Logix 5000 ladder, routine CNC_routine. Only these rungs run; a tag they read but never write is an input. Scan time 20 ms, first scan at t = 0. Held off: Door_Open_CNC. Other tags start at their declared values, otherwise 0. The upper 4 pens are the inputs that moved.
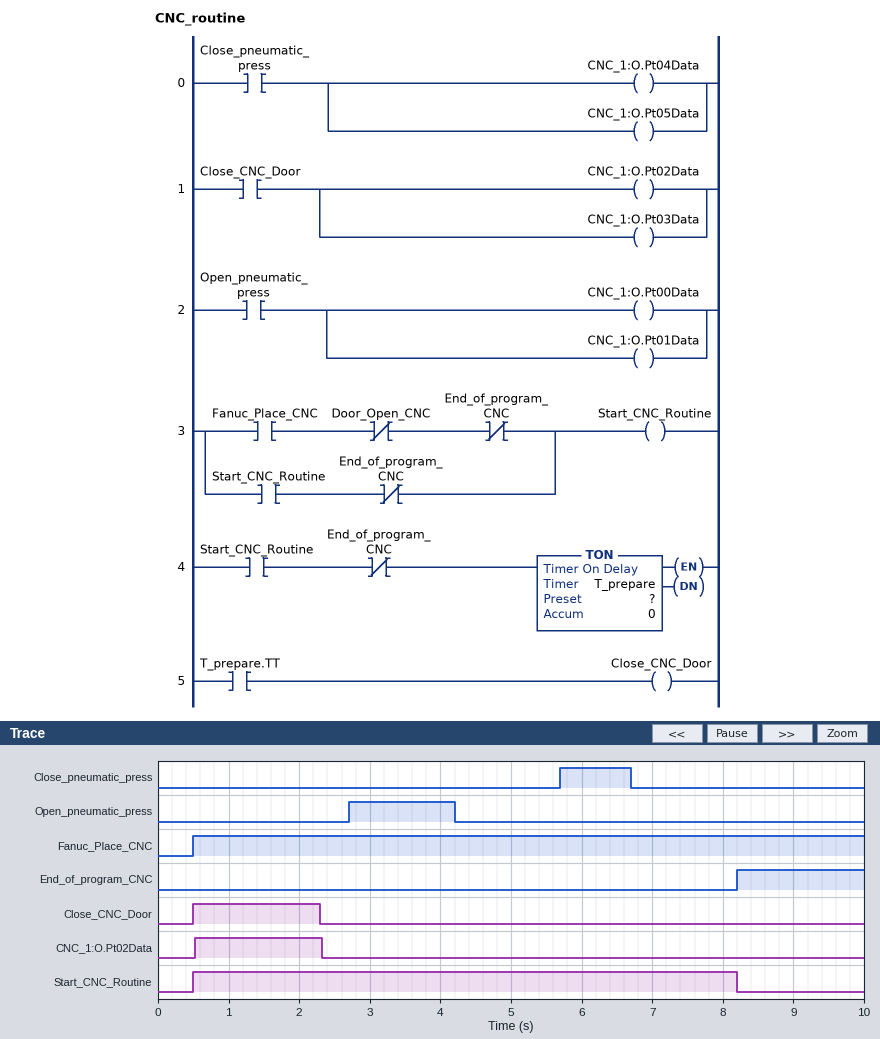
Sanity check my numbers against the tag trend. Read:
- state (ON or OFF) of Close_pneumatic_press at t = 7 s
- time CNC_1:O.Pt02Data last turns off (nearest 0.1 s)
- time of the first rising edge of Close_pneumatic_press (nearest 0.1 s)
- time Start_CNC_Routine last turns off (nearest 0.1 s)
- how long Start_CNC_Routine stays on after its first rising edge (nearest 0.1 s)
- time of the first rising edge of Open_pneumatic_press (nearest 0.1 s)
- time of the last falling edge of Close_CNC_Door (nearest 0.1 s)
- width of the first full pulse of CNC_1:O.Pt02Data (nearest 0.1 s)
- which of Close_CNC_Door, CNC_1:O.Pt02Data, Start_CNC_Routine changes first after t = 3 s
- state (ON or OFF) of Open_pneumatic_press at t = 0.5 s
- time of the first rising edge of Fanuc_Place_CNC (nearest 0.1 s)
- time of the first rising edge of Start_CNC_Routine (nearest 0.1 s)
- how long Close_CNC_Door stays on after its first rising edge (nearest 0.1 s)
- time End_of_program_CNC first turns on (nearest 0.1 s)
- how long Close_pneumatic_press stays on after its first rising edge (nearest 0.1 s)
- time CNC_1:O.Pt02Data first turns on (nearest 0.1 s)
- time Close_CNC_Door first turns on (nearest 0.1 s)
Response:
OFF
2.3 s
5.7 s
8.2 s
7.7 s
2.7 s
2.3 s
1.8 s
Start_CNC_Routine
OFF
0.5 s
0.5 s
1.8 s
8.2 s
1.0 s
0.5 s
0.5 s
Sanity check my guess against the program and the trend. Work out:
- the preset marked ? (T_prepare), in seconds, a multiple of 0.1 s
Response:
1.8 s
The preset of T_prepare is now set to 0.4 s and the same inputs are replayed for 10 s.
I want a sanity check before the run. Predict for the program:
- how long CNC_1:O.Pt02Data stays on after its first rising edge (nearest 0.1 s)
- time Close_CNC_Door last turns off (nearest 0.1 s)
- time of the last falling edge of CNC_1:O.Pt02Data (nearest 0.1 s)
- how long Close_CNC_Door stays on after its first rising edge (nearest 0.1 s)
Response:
0.4 s
0.9 s
0.9 s
0.4 s
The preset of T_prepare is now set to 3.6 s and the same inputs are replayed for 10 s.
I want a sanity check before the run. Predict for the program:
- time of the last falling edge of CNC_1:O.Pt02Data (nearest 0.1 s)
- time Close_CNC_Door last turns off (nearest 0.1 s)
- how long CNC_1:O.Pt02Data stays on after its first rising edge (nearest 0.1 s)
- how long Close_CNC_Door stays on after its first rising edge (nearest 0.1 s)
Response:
4.1 s
4.1 s
3.6 s
3.6 s
